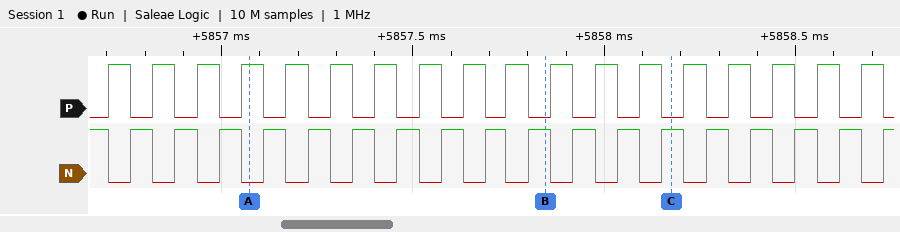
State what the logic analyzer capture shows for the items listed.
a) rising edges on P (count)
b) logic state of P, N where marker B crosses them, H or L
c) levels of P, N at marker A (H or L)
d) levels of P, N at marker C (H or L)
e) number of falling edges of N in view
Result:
18
P=L, N=H
P=H, N=L
P=L, N=H
18
